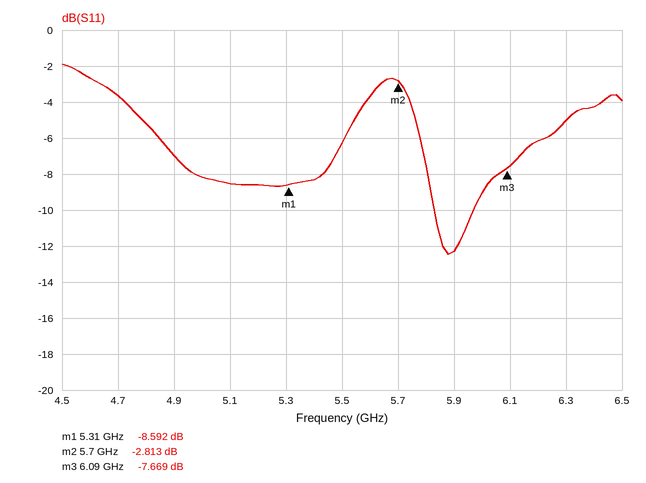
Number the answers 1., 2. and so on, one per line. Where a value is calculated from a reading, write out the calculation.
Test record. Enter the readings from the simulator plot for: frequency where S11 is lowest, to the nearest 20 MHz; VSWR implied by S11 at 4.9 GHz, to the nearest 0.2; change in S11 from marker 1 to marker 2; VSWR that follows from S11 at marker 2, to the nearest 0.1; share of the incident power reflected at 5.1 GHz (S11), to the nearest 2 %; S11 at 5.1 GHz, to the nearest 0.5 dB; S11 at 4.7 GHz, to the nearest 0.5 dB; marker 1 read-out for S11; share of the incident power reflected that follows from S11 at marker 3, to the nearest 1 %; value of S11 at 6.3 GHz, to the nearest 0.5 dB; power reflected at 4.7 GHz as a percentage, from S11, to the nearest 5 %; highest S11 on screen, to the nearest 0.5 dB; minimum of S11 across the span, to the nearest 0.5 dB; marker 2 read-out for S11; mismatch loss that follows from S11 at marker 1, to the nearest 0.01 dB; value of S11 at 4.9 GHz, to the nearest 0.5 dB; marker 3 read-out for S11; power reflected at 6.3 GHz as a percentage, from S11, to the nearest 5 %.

1. 5.88 GHz
2. |Γ| = 10^(-7/20) = 0.4467; VSWR = (1 + 0.4467)/(1 − 0.4467) ≈ 2.6
3. -2.813 − (-8.592) = 5.779 dB
4. (1 + 0.7234)/(1 − 0.7234) ≈ 6.2
5. 10^(-8.5/10) ≈ 14 %
6. -8.5 dB
7. -3.5 dB
8. -8.592 dB
9. 10^(-7.669/10) ≈ 17 %
10. -5.0 dB
11. 10^(-3.5/10) ≈ 45 %
12. -2.0 dB
13. -12.5 dB
14. -2.813 dB
15. −10 log10(1 − 10^(-8.592/10)) ≈ 0.65 dB
16. -7.0 dB
17. -7.669 dB
18. 10^(-5/10) ≈ 31.6 %, so 30 % to the nearest 5 %
